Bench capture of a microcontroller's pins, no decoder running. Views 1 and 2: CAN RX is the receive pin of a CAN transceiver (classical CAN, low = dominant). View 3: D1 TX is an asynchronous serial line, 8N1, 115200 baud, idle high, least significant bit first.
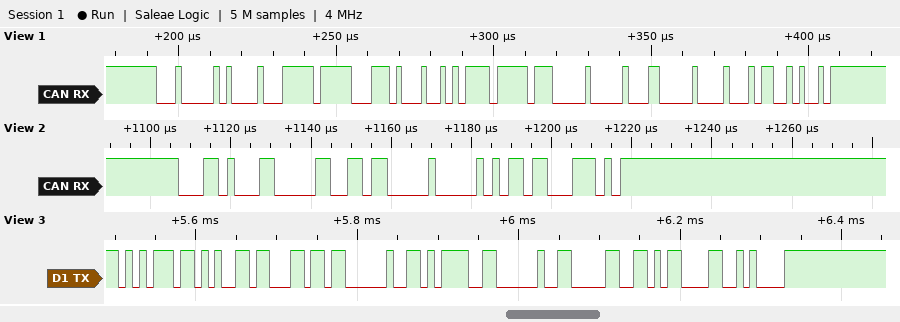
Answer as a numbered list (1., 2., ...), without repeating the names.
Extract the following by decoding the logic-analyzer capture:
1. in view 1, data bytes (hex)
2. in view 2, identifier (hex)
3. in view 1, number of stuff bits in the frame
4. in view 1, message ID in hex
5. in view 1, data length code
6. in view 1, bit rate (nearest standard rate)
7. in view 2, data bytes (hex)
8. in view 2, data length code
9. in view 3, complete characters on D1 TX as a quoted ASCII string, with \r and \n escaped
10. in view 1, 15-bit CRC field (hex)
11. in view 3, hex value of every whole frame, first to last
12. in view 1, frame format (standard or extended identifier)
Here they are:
1. FF CE 89 5E FF 00 06 00
2. 0x1A3
3. 7
4. 0x102
5. 8
6. 500 kbit/s
7. 6C 00
8. 2
9. "uel = 0\r\n"
10. 0x4594
11. 75 65 6C 20 3D 20 30 0D 0A
12. standard
